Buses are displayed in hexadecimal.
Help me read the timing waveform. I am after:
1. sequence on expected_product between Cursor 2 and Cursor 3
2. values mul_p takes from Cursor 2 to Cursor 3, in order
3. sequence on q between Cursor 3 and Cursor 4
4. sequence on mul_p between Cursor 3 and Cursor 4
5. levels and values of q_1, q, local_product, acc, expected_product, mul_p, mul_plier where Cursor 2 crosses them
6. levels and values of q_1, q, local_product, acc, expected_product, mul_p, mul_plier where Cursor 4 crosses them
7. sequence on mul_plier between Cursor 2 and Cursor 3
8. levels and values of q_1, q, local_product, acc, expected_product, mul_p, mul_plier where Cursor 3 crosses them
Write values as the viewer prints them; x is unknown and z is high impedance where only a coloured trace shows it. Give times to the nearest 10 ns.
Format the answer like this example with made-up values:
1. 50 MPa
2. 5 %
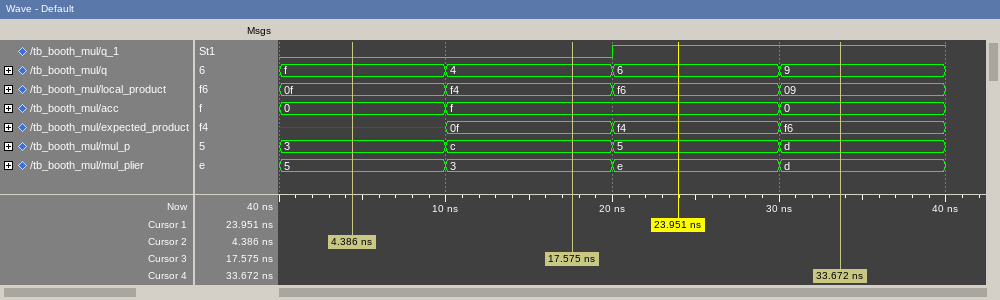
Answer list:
1. x, 0f
2. 3, c
3. 4, 6, 9
4. c, 5, d
5. q_1=0, q=f, local_product=0f, acc=0, expected_product=x, mul_p=3, mul_plier=5
6. q_1=1, q=9, local_product=09, acc=0, expected_product=f6, mul_p=d, mul_plier=d
7. 5, 3
8. q_1=0, q=4, local_product=f4, acc=f, expected_product=0f, mul_p=c, mul_plier=3
